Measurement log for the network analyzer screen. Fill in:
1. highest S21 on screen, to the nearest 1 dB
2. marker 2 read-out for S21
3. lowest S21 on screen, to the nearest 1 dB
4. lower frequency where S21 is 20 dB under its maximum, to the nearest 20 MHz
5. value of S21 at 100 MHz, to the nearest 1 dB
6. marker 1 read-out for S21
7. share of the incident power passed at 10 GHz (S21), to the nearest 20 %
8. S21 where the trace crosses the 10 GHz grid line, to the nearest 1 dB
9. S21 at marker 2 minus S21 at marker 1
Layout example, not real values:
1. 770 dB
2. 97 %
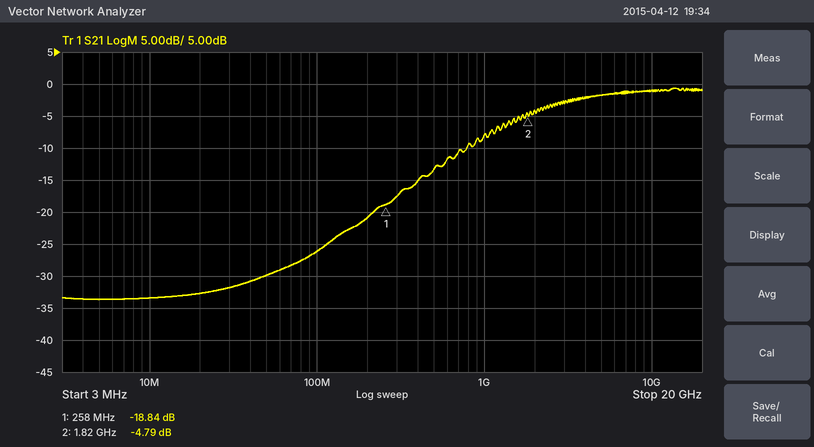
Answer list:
1. -1 dB
2. -4.79 dB
3. -34 dB
4. 200 MHz
5. -26 dB
6. -18.84 dB
7. 80 %
8. -1 dB
9. 14.05 dB
